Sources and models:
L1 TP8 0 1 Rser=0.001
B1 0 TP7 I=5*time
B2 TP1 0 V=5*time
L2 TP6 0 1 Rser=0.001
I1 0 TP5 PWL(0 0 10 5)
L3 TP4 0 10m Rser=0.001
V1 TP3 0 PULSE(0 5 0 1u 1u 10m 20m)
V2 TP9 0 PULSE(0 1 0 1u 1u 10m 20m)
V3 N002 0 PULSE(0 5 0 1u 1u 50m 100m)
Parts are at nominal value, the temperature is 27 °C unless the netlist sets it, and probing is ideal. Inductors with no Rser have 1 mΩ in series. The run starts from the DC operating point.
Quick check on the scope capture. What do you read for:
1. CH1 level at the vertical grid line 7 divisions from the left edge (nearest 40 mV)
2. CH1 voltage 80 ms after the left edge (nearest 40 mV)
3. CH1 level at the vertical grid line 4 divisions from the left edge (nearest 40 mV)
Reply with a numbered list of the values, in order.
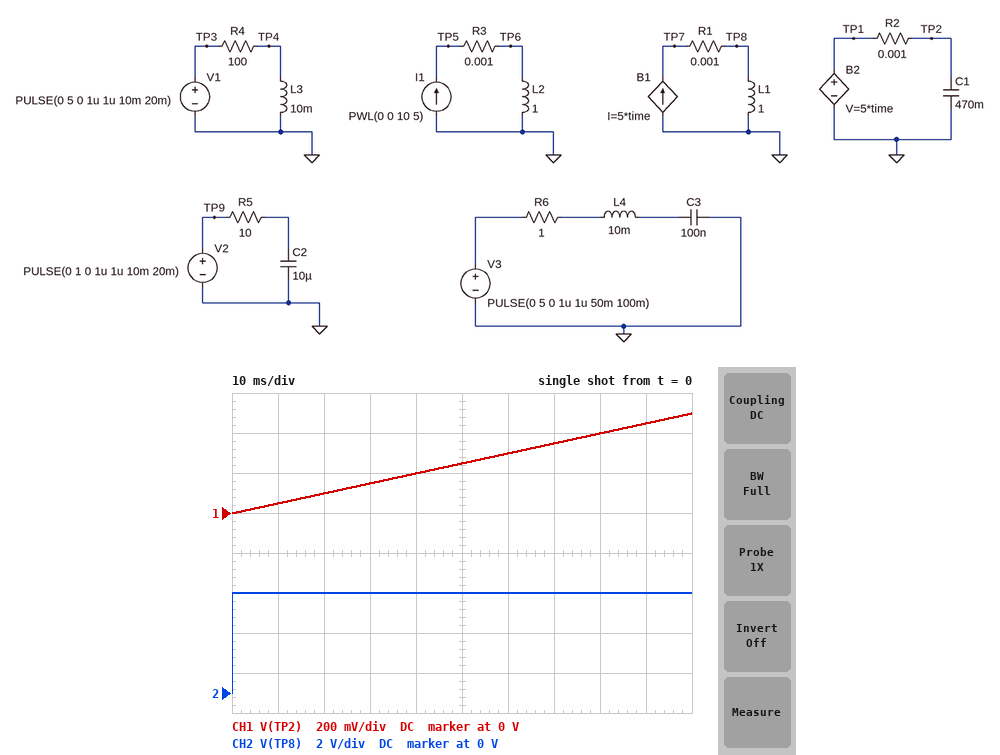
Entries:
1. 360 mV
2. 400 mV
3. 200 mV
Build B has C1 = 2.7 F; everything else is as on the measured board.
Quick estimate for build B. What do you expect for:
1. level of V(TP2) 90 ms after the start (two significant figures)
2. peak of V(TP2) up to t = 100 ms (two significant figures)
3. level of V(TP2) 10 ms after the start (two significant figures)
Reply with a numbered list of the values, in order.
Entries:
1. 440 mV
2. 490 mV
3. 37 mV
